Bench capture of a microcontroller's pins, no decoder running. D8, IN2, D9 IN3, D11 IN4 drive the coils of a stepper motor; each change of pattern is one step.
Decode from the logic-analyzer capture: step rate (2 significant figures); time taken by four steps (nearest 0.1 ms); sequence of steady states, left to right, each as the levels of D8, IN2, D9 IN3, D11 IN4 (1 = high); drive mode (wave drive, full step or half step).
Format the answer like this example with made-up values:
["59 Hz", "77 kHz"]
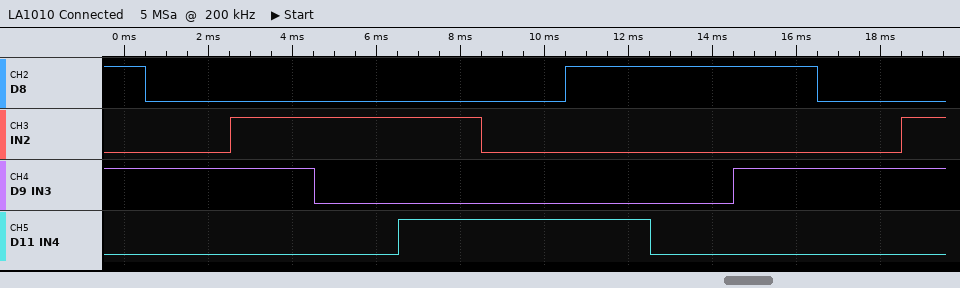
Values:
["500 steps/s", "8.0 ms", "1010 0010 0110 0100 0101 0001 1001 1000 1010 0010 0110", "half step"]
